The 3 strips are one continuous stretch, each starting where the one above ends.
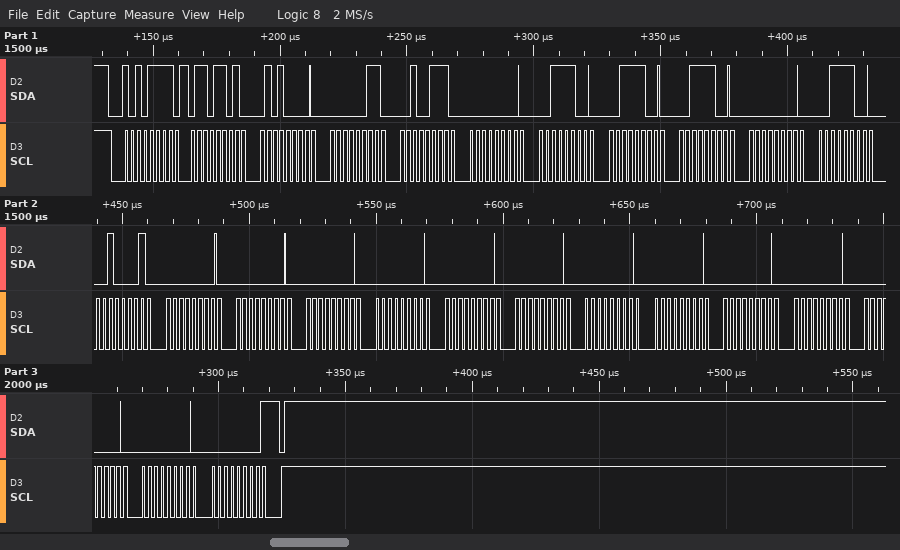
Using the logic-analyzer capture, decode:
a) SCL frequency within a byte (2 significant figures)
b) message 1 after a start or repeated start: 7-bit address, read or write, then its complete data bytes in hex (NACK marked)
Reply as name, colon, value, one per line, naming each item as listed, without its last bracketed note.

SCL frequency within a byte: 400 kHz
message 1 after a start or repeated start: 7-bit address, read or write, then its complete data bytes in hex: 0x57 read: 6D 50 03 27 00 3C 3C 3C 00 3C 21 00 00 00 00 00 00 00 00 00 00 00 00 00 NACK
